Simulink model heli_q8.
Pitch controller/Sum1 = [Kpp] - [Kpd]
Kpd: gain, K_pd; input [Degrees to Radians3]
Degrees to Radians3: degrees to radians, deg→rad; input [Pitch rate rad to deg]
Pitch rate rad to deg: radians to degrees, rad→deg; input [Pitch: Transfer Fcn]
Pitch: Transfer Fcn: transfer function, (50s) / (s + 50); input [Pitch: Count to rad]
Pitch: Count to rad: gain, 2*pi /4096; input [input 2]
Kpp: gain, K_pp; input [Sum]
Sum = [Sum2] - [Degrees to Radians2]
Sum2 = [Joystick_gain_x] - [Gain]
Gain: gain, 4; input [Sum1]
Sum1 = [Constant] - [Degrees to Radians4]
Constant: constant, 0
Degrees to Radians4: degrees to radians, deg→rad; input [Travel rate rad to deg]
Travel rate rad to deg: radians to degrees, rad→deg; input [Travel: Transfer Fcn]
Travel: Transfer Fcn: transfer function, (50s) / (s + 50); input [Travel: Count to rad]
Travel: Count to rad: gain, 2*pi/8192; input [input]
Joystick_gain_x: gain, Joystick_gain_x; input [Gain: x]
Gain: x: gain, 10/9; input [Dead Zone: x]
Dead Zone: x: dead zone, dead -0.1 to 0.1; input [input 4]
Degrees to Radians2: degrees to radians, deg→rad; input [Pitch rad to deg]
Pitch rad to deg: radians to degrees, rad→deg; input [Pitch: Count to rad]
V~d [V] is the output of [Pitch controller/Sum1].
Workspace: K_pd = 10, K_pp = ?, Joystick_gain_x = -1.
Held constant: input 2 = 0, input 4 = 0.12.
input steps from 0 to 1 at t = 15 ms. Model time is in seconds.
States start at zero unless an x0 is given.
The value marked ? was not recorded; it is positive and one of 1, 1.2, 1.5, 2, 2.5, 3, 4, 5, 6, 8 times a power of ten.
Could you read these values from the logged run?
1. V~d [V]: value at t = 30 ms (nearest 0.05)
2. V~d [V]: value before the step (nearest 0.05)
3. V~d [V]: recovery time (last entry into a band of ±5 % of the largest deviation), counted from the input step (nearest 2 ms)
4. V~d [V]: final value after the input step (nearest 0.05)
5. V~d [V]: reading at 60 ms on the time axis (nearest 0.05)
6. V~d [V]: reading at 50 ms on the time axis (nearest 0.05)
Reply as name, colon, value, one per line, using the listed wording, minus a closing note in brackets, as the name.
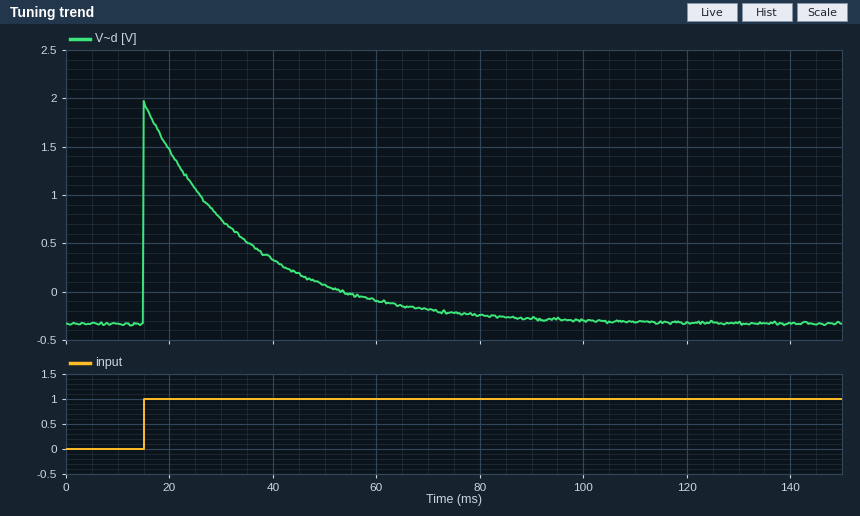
V~d [V]: value at t = 30 ms: 0.75
V~d [V]: value before the step: -0.35
V~d [V]: recovery time (last entry into a band of ±5 % of the largest deviation), counted from the input step: 60 ms
V~d [V]: final value after the input step: -0.35
V~d [V]: reading at 60 ms on the time axis: -0.10
V~d [V]: reading at 50 ms on the time axis: 0.05
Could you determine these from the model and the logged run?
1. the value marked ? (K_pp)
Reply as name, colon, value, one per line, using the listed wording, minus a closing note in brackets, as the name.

the value marked ?: 15
